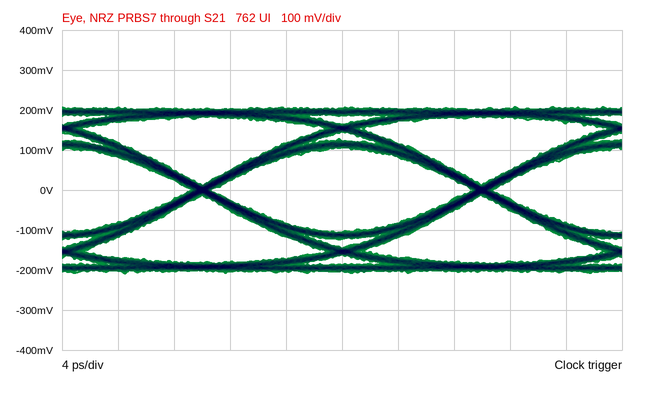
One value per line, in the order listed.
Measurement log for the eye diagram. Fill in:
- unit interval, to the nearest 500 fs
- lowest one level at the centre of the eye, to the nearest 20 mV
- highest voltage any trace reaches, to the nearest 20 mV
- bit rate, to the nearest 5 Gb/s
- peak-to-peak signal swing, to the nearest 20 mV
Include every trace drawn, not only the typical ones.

20.0 ps
100 mV
200 mV
50 Gb/s
420 mV
